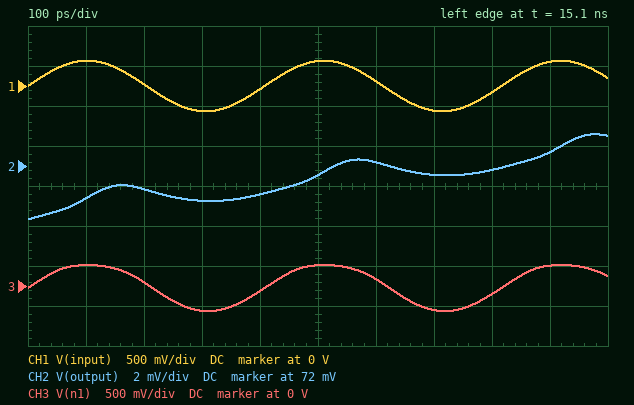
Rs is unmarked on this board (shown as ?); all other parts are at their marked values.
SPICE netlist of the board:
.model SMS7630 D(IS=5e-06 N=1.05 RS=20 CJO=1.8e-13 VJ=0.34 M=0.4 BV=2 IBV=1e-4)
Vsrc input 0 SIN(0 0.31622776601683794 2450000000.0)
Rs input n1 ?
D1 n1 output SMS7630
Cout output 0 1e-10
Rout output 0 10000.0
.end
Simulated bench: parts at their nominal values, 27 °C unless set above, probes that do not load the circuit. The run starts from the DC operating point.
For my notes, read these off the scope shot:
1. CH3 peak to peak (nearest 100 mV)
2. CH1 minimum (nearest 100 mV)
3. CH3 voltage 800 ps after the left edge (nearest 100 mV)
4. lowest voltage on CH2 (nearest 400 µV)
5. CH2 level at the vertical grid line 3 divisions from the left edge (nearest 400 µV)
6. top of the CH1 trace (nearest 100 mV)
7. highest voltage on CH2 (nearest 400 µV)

600 mV
-300 mV
-100 mV
69.2 mV
70.4 mV
300 mV
73.6 mV
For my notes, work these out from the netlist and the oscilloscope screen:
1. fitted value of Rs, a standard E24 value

33 Ω
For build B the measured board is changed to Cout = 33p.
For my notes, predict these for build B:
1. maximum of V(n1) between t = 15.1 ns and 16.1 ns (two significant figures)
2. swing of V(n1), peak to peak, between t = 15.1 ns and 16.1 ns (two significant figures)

290 mV
600 mV
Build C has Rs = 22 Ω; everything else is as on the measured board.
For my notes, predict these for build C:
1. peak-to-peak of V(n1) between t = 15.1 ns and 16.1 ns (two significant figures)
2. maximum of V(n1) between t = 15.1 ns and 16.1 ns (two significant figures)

590 mV
280 mV
